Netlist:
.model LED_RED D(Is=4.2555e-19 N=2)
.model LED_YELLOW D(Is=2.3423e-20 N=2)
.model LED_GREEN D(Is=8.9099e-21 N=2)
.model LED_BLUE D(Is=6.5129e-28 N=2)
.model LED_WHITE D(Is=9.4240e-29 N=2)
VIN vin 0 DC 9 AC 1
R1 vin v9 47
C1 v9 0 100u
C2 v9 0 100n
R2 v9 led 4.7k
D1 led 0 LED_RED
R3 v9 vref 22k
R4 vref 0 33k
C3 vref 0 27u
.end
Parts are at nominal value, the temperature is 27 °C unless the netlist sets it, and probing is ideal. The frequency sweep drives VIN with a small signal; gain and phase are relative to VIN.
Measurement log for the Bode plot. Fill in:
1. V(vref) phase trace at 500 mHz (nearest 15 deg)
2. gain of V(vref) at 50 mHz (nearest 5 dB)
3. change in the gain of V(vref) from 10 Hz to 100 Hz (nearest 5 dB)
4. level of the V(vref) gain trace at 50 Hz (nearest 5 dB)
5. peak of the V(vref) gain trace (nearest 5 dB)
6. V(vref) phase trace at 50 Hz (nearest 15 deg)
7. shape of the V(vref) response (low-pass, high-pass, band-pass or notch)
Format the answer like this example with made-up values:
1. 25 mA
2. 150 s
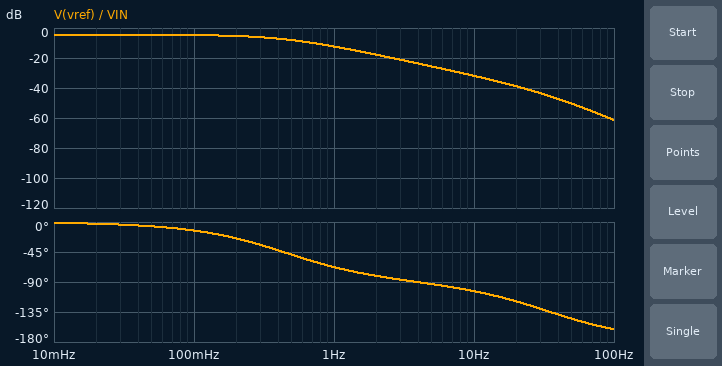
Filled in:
1. -45 deg
2. -5 dB
3. -30 dB
4. -50 dB
5. -5 dB
6. -150 deg
7. low-pass
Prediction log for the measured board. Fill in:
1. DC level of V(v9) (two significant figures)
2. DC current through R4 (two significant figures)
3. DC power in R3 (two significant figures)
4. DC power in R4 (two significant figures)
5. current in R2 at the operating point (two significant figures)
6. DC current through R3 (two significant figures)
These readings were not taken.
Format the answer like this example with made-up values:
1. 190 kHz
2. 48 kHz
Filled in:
1. 8.9 V
2. 160 µA
3. 580 µW
4. 870 µW
5. 1.5 mA
6. 160 µA
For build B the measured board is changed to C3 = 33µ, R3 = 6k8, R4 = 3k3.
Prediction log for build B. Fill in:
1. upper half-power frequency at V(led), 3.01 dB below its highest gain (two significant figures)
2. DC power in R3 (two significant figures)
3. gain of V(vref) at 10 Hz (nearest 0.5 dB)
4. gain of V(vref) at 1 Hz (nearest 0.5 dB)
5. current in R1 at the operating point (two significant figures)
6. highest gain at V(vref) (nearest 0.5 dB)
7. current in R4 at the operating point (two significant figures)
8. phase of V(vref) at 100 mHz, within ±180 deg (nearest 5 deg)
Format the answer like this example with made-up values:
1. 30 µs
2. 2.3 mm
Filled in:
1. 34 Hz
2. 5.3 mW
3. -23.5 dB
4. -10.5 dB
5. 2.4 mA
6. -10.0 dB
7. 880 µA
8. -5 deg
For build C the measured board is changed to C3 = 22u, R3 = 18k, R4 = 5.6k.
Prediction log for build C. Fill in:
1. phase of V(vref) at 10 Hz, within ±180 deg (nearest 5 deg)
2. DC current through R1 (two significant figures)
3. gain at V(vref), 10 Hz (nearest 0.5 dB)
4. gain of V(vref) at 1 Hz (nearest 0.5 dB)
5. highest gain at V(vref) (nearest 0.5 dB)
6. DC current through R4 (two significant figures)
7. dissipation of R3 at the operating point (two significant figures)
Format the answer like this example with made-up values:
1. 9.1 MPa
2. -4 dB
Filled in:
1. -95 deg
2. 1.9 mA
3. -28.5 dB
4. -14.0 dB
5. -12.5 dB
6. 380 µA
7. 2.6 mW
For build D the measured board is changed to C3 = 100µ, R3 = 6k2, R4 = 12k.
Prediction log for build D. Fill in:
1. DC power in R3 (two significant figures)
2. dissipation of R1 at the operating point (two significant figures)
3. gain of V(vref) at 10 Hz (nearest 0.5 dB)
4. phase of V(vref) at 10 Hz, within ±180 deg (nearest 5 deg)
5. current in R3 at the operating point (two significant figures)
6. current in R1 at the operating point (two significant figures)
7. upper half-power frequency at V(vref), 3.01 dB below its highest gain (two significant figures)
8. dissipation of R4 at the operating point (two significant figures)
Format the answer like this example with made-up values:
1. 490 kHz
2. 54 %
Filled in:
1. 1.5 mW
2. 190 µW
3. -32.5 dB
4. -105 deg
5. 490 µA
6. 2.0 mA
7. 390 mHz
8. 2.9 mW
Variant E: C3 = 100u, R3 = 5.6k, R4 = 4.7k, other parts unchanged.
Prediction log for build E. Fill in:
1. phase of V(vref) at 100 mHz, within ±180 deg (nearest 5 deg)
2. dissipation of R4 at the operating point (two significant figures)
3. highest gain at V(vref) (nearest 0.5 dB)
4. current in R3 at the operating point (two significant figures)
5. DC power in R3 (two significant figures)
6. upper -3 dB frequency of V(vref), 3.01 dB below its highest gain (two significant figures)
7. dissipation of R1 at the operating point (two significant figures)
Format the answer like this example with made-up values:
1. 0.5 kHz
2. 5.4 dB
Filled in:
1. -10 deg
2. 3.5 mW
3. -7.0 dB
4. 860 µA
5. 4.2 mW
6. 620 mHz
7. 260 µW
